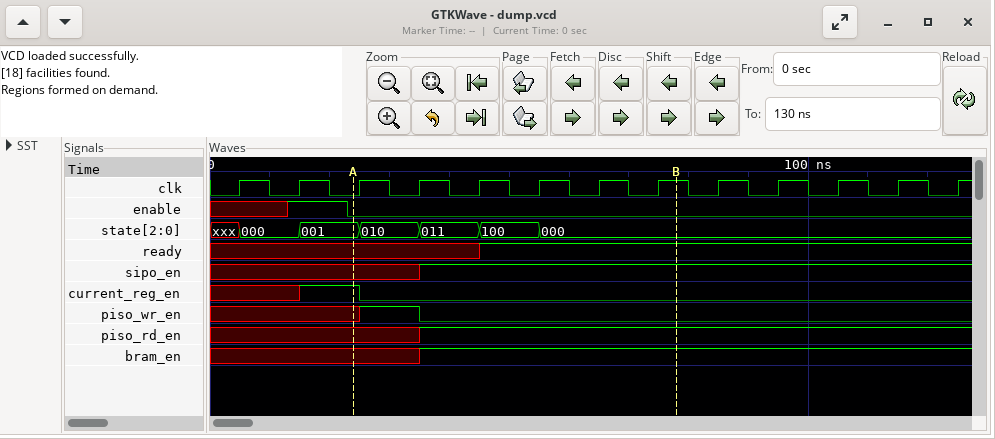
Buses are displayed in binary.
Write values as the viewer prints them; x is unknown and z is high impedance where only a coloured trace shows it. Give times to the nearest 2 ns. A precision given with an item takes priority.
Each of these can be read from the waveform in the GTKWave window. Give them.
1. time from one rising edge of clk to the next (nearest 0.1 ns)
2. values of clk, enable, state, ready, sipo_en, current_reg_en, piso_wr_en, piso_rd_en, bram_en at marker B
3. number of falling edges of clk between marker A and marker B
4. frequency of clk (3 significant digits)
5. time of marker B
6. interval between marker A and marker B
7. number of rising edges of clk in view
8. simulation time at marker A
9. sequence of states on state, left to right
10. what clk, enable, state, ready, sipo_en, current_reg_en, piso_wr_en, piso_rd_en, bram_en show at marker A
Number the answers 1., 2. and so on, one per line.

1. 10 ns
2. clk=1, enable=0, state=000, ready=1, sipo_en=1, current_reg_en=0, piso_wr_en=0, piso_rd_en=1, bram_en=1
3. 5
4. 100 MHz
5. 78 ns
6. 54 ns
7. 13
8. 24 ns
9. xxx, 000, 001, 010, 011, 100, 000
10. clk=0, enable=0, state=001, ready=x, sipo_en=x, current_reg_en=1, piso_wr_en=x, piso_rd_en=x, bram_en=x
